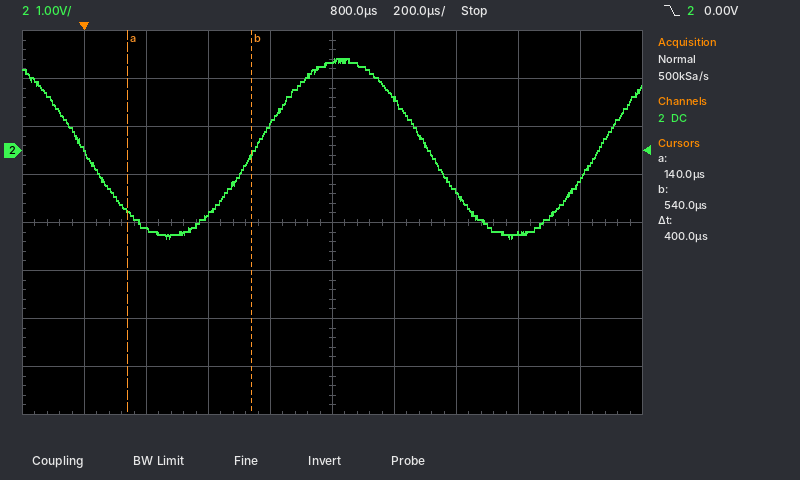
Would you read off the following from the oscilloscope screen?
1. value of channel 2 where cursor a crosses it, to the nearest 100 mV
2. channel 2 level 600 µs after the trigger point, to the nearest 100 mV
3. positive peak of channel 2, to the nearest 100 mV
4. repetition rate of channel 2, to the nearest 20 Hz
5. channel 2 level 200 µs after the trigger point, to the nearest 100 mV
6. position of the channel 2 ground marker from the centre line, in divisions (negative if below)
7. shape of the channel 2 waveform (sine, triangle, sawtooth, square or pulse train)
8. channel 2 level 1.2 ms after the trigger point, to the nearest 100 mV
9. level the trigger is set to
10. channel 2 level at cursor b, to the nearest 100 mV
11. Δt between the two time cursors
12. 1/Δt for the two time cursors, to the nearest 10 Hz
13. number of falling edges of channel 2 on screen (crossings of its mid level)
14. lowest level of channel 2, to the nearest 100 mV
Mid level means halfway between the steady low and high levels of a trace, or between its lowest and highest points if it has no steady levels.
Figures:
-1.3 V
600 mV
1.9 V
900 Hz
-1.6 V
+1.5 div
sine
-900 mV
0.00 V
-100 mV
400 µs
2.50 kHz
2
-1.8 V
